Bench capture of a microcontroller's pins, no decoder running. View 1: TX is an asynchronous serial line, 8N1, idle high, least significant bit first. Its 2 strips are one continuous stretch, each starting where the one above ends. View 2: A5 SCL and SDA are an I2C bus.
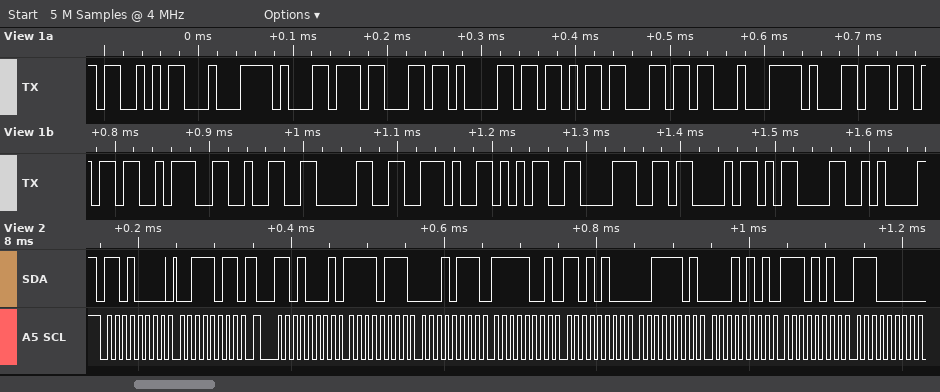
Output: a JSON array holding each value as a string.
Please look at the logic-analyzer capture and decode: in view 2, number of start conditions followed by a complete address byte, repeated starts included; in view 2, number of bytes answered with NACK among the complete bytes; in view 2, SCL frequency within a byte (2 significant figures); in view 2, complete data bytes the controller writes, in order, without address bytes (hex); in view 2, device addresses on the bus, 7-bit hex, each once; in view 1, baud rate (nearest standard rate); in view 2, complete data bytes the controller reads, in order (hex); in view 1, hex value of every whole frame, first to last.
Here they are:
["2", "0", "100 kHz", "3B", "0x68", "115200 baud", "F7 17 F9 D4 3D 15 EA E0", "53 C4 B1 63 61 6B 6C C4 B1 6B 3A 32 30 2E 35 38 43 0D 0A"]
